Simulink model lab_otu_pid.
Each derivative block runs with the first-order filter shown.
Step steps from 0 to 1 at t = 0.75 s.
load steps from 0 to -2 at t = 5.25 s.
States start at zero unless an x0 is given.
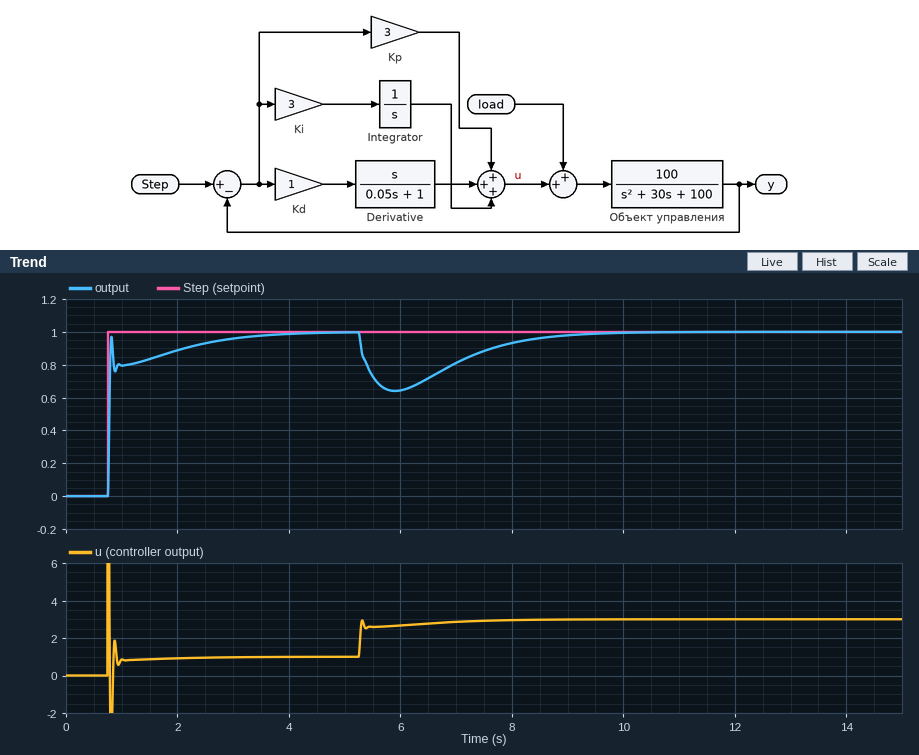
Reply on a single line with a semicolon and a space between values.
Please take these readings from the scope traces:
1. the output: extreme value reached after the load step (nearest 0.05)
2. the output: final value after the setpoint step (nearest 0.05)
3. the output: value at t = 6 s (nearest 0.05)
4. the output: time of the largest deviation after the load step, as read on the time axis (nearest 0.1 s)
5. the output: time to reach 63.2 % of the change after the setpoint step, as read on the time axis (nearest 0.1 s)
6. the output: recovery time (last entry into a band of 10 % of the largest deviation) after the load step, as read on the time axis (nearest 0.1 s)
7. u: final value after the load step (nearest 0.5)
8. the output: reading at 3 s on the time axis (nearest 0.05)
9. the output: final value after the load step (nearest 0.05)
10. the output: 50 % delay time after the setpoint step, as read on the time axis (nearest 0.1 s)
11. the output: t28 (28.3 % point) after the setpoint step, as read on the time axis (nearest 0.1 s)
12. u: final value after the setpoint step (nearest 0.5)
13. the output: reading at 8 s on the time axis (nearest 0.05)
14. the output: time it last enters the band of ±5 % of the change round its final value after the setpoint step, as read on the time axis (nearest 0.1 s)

0.65; 1.00; 0.65; 5.9 s; 0.8 s; 8.6 s; 3.0; 0.95; 1.00; 0.8 s; 0.8 s; 1.0; 0.95; 2.8 s
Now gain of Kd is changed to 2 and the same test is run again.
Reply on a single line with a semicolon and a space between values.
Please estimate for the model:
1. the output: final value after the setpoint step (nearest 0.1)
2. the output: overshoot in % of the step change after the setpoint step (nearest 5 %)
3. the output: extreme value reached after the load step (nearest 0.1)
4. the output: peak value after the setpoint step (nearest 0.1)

1.0; 15 %; 0.7; 1.1
